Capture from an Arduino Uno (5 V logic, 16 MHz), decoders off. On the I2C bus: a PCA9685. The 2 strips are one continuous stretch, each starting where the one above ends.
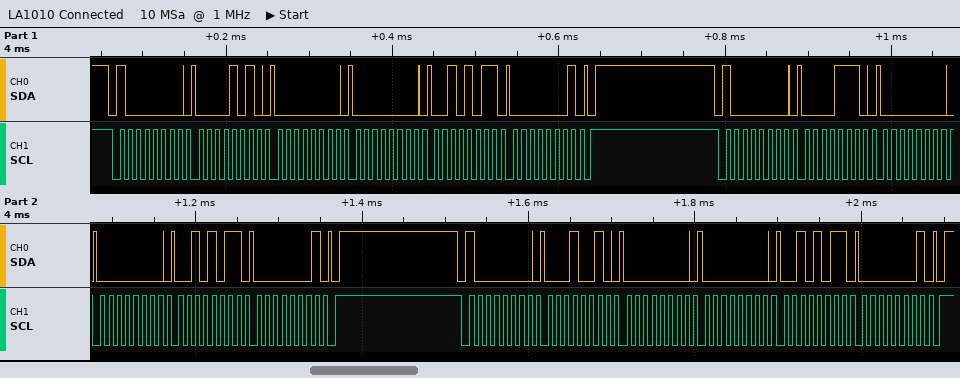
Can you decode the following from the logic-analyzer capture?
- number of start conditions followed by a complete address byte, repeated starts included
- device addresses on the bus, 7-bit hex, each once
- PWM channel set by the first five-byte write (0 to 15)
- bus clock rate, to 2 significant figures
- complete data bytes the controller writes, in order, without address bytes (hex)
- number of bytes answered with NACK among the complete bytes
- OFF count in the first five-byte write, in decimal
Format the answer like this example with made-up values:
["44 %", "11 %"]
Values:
["3", "0x40", "1", "100 kHz", "0A 00 00 2B 01 0E 00 00 2B 01 12 00 00 2B 01", "0", "299"]
